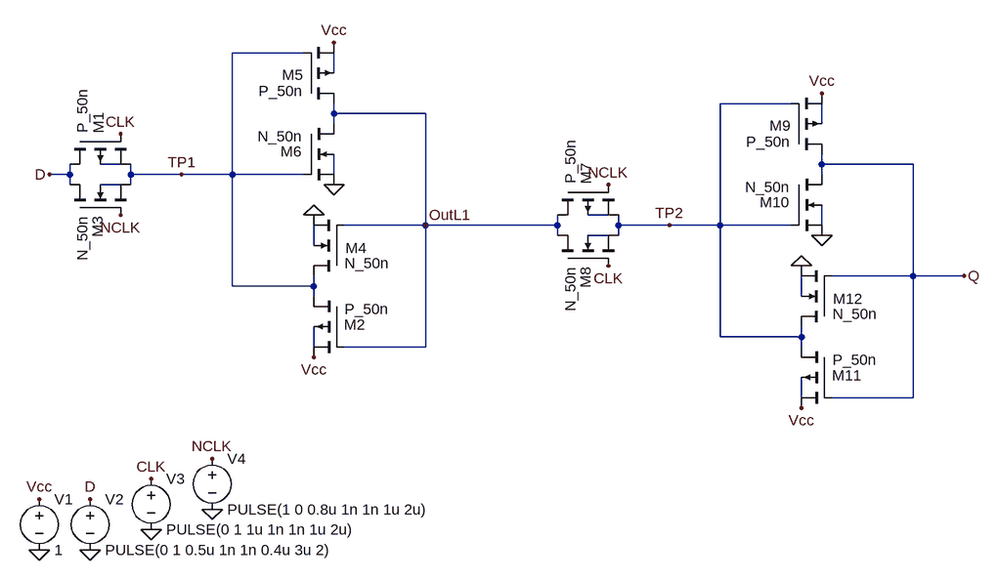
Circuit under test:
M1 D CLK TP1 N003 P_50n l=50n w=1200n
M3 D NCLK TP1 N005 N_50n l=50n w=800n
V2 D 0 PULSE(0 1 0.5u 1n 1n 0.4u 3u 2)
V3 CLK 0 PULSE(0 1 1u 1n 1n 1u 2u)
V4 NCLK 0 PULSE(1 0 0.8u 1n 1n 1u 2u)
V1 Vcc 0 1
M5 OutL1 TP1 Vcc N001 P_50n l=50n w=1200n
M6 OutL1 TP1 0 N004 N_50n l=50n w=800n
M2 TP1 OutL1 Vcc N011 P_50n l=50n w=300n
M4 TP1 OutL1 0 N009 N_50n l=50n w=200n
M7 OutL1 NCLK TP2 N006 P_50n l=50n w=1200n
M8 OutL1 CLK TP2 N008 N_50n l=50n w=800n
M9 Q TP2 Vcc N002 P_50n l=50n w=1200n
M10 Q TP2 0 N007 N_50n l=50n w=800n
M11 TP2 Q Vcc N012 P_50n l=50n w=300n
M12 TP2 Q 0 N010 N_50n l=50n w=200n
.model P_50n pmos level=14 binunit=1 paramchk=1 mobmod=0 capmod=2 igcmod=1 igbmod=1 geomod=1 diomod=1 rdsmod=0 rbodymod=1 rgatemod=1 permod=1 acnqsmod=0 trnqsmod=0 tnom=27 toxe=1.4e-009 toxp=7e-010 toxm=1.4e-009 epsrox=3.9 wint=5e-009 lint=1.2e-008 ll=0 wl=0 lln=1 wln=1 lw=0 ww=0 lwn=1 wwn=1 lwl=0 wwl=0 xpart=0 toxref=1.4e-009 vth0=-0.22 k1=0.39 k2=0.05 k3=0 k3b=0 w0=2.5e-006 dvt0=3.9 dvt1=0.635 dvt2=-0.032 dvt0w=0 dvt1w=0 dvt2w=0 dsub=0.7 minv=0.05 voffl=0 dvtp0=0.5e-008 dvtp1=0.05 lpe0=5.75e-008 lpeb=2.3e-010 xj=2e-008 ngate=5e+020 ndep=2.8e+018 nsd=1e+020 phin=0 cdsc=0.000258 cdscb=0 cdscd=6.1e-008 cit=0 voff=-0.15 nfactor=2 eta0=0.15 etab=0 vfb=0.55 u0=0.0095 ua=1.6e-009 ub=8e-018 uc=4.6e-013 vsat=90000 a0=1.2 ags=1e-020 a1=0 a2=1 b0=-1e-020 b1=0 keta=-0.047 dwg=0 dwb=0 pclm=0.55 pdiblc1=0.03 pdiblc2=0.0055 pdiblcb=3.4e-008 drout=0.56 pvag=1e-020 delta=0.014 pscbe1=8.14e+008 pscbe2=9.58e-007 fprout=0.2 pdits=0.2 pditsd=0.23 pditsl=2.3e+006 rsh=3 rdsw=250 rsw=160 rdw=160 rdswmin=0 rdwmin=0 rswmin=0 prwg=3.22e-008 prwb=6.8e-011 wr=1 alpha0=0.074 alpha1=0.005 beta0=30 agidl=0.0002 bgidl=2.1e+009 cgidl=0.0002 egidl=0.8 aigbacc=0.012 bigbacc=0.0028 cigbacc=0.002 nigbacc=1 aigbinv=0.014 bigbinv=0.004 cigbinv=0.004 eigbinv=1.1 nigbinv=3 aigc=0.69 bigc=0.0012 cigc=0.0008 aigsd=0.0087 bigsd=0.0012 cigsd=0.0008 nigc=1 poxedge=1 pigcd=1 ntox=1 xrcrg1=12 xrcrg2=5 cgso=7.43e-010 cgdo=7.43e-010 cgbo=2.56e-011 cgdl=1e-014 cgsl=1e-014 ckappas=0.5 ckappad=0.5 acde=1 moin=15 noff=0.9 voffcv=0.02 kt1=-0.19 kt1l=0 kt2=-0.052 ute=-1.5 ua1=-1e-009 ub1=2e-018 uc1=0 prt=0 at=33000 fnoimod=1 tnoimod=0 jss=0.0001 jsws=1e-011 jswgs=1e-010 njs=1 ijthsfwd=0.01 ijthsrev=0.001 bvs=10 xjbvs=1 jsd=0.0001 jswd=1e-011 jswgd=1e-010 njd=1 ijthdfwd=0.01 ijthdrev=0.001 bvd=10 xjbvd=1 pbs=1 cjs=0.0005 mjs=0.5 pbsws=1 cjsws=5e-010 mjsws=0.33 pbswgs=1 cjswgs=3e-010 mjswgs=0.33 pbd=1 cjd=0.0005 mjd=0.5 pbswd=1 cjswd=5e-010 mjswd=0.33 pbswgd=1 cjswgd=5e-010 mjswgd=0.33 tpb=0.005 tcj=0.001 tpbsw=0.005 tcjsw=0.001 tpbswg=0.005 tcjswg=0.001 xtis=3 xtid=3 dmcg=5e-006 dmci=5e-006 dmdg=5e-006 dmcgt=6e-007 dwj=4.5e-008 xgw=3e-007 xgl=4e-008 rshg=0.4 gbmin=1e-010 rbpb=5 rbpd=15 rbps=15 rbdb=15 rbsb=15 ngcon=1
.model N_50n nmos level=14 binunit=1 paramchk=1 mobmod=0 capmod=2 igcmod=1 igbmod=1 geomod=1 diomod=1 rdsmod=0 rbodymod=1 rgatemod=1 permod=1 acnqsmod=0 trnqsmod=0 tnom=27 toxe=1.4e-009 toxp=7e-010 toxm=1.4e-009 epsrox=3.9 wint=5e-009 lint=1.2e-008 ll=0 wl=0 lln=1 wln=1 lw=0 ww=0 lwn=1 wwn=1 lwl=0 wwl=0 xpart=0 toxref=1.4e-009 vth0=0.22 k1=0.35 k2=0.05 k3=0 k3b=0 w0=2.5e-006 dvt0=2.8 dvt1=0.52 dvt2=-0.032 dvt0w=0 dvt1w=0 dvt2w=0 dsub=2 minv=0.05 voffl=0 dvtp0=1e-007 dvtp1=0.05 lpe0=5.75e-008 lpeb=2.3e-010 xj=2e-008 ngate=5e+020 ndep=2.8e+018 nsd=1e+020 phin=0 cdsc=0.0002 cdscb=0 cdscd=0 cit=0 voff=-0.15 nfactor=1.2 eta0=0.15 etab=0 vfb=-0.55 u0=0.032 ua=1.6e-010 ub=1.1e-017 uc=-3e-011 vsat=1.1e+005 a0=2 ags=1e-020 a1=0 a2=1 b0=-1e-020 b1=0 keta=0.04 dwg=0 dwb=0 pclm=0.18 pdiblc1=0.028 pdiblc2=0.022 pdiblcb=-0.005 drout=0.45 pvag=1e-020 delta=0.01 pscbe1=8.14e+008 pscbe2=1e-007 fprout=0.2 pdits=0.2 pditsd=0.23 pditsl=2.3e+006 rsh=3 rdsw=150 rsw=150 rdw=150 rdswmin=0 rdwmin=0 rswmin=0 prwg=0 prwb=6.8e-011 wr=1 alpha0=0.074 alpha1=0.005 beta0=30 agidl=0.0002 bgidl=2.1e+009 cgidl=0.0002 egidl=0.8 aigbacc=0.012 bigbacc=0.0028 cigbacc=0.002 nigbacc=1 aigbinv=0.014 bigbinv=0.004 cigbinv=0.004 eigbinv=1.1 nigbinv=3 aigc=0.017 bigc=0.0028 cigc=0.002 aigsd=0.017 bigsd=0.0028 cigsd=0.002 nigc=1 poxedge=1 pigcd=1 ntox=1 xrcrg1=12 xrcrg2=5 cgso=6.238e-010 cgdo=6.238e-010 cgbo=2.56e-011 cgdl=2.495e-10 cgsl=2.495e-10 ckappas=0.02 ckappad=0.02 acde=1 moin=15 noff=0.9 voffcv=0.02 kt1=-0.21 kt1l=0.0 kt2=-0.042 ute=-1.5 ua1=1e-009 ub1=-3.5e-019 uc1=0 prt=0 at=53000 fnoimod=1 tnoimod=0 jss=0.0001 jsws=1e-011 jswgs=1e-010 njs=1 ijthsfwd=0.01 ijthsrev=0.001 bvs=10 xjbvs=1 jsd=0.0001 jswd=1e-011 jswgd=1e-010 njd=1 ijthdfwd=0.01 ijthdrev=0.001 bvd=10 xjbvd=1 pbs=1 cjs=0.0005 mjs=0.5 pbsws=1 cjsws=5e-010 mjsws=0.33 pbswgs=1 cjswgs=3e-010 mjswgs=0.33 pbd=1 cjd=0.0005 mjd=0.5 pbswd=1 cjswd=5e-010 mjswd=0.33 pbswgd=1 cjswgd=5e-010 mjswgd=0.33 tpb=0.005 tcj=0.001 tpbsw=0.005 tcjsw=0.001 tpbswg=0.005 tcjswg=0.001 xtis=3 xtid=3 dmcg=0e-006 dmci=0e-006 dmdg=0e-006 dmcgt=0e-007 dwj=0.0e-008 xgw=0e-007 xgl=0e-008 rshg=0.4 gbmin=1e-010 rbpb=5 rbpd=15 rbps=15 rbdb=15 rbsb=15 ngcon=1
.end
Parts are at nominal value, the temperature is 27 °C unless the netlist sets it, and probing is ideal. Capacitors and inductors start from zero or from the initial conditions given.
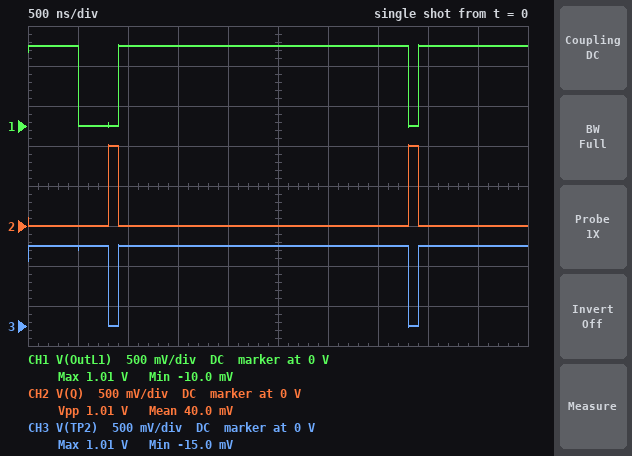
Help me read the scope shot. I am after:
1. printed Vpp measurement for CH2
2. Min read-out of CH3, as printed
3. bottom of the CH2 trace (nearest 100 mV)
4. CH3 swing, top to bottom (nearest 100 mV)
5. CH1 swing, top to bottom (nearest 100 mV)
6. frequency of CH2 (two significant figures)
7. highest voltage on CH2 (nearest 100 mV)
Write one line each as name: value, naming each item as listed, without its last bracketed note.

printed Vpp measurement for CH2: 1.01 V
Min read-out of CH3, as printed: -15.0 mV
bottom of the CH2 trace: 0 V
CH3 swing, top to bottom: 1.0 V
CH1 swing, top to bottom: 1.0 V
frequency of CH2: 330 kHz
highest voltage on CH2: 1.0 V
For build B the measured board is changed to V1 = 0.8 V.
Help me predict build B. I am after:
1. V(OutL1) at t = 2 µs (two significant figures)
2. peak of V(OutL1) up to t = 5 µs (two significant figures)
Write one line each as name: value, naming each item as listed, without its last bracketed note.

V(OutL1) at t = 2 µs: 800 mV
peak of V(OutL1) up to t = 5 µs: 810 mV
